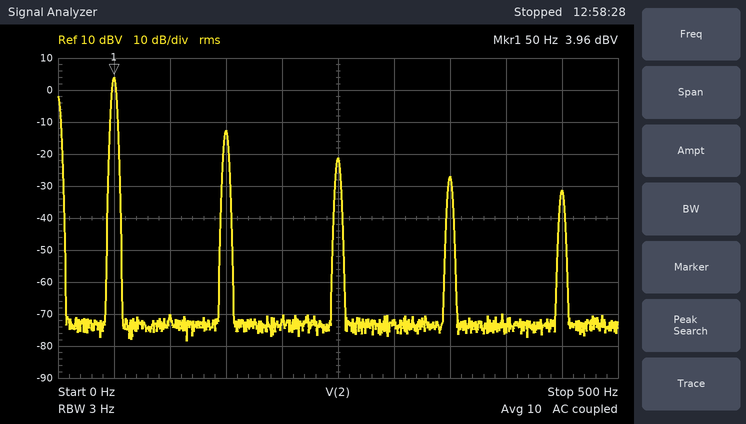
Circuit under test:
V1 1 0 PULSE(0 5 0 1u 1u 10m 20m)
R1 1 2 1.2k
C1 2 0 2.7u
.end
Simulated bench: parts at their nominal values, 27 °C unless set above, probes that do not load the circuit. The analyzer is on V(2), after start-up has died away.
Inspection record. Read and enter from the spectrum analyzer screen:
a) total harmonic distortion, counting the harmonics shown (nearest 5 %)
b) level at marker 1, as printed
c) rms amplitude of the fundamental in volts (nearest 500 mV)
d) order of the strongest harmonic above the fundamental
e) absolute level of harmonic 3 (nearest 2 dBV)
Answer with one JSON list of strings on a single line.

["15 %", "3.96 dBV", "1.5 V", "3", "-12 dBV"]
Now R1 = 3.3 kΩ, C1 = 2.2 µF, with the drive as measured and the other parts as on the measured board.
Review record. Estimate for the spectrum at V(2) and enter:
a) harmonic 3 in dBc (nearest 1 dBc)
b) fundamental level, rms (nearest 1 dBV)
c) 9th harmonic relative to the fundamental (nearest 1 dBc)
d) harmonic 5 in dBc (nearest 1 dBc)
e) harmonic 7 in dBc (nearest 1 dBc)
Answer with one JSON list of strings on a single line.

["-18 dBc", "-1 dBV", "-37 dBc", "-27 dBc", "-33 dBc"]
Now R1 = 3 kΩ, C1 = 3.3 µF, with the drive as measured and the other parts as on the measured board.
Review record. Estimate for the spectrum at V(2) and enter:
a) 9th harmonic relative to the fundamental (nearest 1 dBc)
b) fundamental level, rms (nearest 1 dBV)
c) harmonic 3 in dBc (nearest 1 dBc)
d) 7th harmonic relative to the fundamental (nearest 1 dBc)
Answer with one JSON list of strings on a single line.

["-38 dBc", "-3 dBV", "-19 dBc", "-33 dBc"]
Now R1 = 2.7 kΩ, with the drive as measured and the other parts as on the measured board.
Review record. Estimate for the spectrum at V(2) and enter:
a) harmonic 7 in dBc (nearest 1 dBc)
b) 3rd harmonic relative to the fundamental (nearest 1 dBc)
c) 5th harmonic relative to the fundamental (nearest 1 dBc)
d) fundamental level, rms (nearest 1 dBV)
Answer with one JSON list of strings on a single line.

["-33 dBc", "-18 dBc", "-27 dBc", "-1 dBV"]
